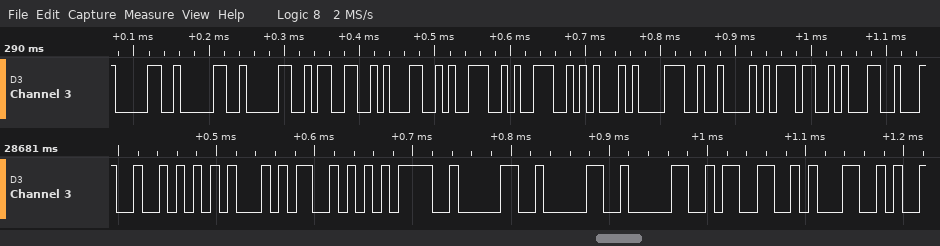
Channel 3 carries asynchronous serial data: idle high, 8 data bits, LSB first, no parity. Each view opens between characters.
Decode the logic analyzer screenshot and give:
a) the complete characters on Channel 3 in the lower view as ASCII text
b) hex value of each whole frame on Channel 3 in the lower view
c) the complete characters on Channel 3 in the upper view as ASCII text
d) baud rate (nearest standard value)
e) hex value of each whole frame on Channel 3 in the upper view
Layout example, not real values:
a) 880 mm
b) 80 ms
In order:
a) "RES=00031"
b) 52, 45, 53, 3D, 30, 30, 30, 33, 31
c) "0003199E8B71"
d) 115200 baud
e) 30, 30, 30, 33, 31, 39, 39, 45, 38, 42, 37, 31
